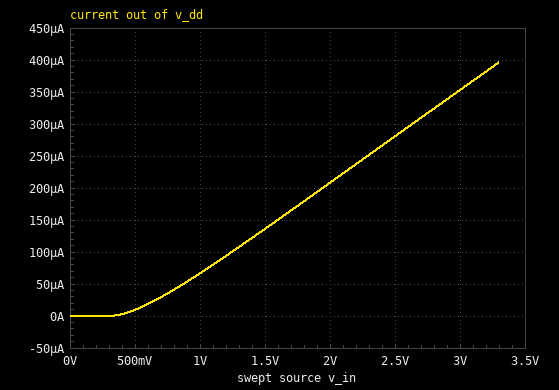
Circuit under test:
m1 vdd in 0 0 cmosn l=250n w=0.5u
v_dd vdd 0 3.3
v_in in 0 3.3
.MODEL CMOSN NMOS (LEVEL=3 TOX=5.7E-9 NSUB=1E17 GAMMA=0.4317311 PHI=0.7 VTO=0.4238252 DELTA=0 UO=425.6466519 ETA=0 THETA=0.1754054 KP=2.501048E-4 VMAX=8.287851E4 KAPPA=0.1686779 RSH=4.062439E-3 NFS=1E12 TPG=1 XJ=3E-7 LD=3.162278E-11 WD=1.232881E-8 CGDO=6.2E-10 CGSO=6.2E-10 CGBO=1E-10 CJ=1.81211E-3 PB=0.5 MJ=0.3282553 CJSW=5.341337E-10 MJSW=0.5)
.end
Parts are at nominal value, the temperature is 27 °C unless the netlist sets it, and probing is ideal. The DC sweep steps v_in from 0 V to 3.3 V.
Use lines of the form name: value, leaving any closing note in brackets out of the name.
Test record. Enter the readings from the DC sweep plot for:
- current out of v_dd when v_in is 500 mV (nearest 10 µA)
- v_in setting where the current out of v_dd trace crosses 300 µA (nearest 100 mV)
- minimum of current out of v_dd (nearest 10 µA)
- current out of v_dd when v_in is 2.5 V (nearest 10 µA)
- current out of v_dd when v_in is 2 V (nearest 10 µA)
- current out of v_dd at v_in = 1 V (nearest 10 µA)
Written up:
current out of v_dd when v_in is 500 mV: 10 µA
v_in setting where the current out of v_dd trace crosses 300 µA: 2.6 V
minimum of current out of v_dd: 0 A
current out of v_dd when v_in is 2.5 V: 280 µA
current out of v_dd when v_in is 2 V: 210 µA
current out of v_dd at v_in = 1 V: 70 µA
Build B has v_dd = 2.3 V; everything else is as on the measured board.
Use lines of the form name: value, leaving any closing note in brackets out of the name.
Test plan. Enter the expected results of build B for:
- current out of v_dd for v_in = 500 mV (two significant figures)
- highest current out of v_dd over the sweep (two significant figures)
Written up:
current out of v_dd for v_in = 500 mV: 9.0 µA
highest current out of v_dd over the sweep: 360 µA
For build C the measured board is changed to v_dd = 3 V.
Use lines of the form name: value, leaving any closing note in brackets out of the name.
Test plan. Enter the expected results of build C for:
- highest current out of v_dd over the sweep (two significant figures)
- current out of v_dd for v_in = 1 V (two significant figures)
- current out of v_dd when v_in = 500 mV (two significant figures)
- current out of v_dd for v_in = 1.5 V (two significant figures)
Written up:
highest current out of v_dd over the sweep: 390 µA
current out of v_dd for v_in = 1 V: 65 µA
current out of v_dd when v_in = 500 mV: 9.5 µA
current out of v_dd for v_in = 1.5 V: 130 µA
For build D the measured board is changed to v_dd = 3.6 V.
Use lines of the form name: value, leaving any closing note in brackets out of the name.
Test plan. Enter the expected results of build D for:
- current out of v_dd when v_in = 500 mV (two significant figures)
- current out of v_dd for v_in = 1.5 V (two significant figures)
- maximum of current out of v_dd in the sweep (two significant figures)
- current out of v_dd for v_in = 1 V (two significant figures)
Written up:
current out of v_dd when v_in = 500 mV: 9.9 µA
current out of v_dd for v_in = 1.5 V: 140 µA
maximum of current out of v_dd in the sweep: 410 µA
current out of v_dd for v_in = 1 V: 68 µA
